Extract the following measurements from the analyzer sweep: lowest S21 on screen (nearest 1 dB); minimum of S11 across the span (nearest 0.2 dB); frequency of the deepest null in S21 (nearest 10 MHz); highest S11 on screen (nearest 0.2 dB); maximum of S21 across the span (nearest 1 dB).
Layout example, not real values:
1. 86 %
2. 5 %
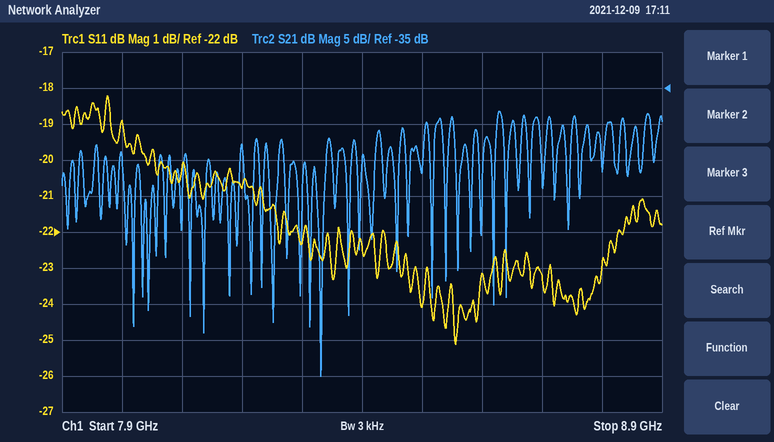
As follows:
1. -75 dB
2. -25.2 dB
3. 8.33 GHz
4. -18.2 dB
5. -38 dB
